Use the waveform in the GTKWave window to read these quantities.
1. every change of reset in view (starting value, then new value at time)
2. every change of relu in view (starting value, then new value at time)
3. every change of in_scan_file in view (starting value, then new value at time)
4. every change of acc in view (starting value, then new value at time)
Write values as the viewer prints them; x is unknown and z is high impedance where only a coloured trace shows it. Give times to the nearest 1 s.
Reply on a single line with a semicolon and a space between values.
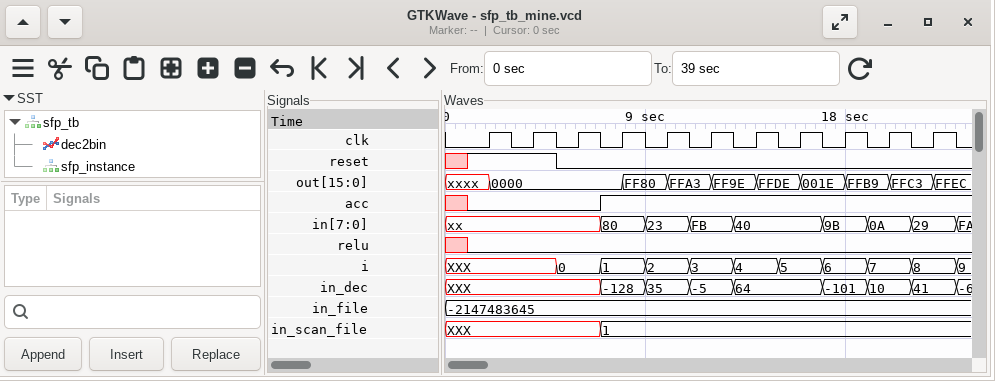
x, 1 at 1 s, 0 at 5 s; x, 0 at 1 s; XXX, 1 at 7 s; x, 0 at 1 s, 1 at 7 s
